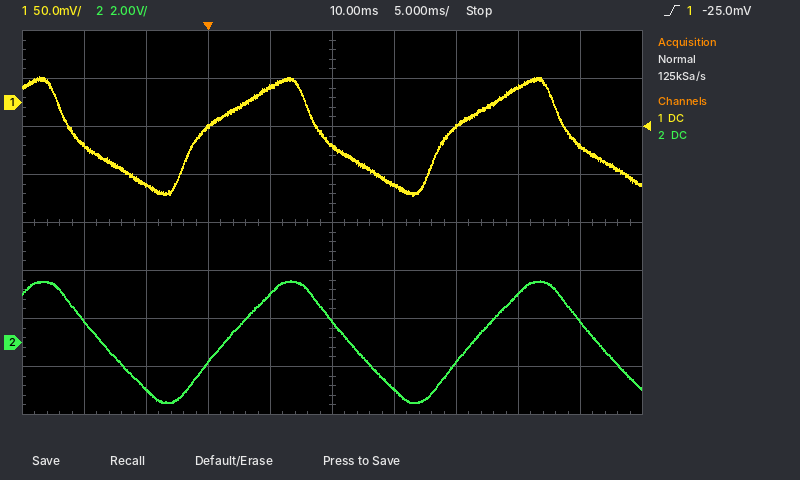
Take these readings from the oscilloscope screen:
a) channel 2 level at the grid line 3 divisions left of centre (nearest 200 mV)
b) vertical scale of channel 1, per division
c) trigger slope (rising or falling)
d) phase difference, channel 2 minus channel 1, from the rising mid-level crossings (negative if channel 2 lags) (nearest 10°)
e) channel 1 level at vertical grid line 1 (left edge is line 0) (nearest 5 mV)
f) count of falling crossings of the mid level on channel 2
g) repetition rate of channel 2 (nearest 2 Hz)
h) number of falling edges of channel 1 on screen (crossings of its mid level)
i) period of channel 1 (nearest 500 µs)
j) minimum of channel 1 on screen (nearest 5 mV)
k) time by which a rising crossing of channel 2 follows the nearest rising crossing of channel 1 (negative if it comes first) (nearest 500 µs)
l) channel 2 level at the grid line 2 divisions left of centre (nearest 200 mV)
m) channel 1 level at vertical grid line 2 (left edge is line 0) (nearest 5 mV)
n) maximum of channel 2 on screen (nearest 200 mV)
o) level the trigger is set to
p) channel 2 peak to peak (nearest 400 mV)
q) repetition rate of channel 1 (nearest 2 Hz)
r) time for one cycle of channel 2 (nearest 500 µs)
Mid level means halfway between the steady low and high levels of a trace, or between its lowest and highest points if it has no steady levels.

-2.0 V
50 mV
rising
-40°
-45 mV
3
50 Hz
3
20.0 ms
-95 mV
+2.0 ms
-800 mV
-85 mV
2.6 V
-25.0 mV
5.2 V
50 Hz
20.0 ms
